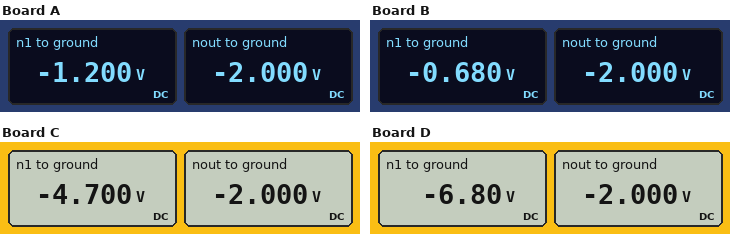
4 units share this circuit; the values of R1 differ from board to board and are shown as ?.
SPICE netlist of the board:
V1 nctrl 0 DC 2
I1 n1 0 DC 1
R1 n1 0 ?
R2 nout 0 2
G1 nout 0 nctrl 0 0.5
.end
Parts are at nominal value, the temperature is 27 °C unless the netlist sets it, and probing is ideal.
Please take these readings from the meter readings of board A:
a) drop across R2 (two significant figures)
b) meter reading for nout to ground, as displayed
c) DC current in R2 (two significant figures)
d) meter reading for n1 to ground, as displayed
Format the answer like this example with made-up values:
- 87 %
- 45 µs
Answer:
- 2.0 V
- -2.000 V
- 1.0 A
- -1.200 V
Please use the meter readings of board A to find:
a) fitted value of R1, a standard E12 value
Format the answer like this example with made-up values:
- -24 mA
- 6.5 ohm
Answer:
- 1.2 Ω
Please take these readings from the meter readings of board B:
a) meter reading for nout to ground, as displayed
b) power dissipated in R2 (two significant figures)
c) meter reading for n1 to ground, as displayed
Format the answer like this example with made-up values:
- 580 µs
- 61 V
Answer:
- -2.000 V
- 2.0 W
- -0.680 V
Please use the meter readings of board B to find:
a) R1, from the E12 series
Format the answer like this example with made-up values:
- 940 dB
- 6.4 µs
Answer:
- 0.68 Ω
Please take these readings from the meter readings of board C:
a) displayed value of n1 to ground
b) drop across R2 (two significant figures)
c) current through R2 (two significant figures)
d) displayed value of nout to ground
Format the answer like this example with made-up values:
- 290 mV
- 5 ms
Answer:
- -4.700 V
- 2.0 V
- 1.0 A
- -2.000 V
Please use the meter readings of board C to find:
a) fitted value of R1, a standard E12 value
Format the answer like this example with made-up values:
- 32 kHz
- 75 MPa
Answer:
- 4.7 Ω
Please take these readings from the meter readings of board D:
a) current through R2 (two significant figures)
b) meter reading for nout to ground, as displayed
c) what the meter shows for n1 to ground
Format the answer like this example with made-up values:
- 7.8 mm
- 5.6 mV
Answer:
- 1.0 A
- -2.000 V
- -6.80 V
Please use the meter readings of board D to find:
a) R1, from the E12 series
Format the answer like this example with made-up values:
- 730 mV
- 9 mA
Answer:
- 6.8 Ω
